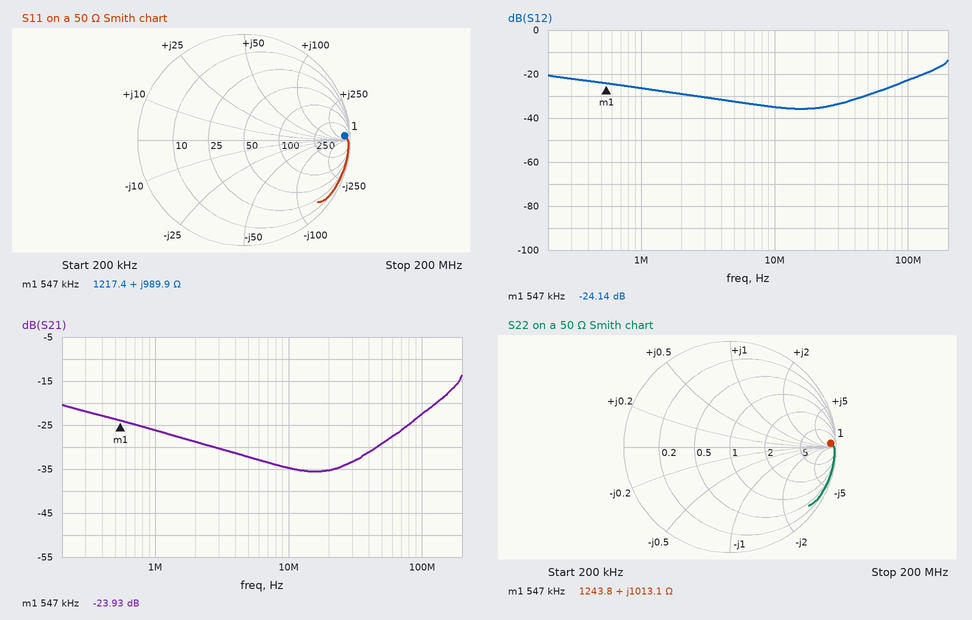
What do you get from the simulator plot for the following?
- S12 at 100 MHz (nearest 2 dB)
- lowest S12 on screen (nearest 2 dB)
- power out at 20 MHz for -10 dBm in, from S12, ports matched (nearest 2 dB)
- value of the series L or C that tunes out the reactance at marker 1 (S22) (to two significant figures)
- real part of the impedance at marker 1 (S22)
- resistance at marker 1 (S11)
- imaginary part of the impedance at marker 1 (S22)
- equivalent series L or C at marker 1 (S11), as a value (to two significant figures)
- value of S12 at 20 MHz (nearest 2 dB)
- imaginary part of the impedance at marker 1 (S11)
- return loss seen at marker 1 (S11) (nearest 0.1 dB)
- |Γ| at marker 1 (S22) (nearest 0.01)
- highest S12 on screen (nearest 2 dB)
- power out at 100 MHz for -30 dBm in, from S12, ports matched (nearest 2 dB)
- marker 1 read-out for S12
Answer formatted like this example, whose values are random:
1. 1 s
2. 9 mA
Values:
1. -22 dB
2. -36 dB
3. -46 dBm
4. 290 pF
5. 1243.8 Ω
6. 1217.4 Ω
7. +1013.1 Ω
8. 290 µH
9. -36 dB
10. +989.9 Ω
11. 0.4 dB
12. 0.95
13. -14 dB
14. -52 dBm
15. -24.14 dB
